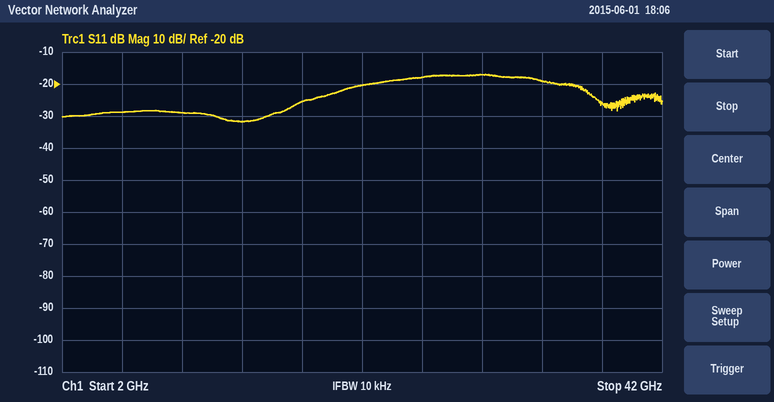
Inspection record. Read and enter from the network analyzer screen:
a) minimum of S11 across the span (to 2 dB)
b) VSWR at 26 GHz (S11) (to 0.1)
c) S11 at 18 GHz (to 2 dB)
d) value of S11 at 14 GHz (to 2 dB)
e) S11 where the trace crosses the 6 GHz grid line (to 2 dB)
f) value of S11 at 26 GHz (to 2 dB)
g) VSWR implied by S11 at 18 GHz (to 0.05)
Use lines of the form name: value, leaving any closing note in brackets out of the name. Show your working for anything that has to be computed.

minimum of S11 across the span: -32 dB
VSWR at 26 GHz (S11): |Γ| = 10^(-18/20) = 0.1259; VSWR = (1 + 0.1259)/(1 − 0.1259) ≈ 1.3
S11 at 18 GHz: -26 dB
value of S11 at 14 GHz: -32 dB
S11 where the trace crosses the 6 GHz grid line: -28 dB
value of S11 at 26 GHz: -18 dB
VSWR implied by S11 at 18 GHz: |Γ| = 10^(-26/20) = 0.0501; VSWR = (1 + 0.0501)/(1 − 0.0501) ≈ 1.11, so 1.10 to the nearest 0.05
